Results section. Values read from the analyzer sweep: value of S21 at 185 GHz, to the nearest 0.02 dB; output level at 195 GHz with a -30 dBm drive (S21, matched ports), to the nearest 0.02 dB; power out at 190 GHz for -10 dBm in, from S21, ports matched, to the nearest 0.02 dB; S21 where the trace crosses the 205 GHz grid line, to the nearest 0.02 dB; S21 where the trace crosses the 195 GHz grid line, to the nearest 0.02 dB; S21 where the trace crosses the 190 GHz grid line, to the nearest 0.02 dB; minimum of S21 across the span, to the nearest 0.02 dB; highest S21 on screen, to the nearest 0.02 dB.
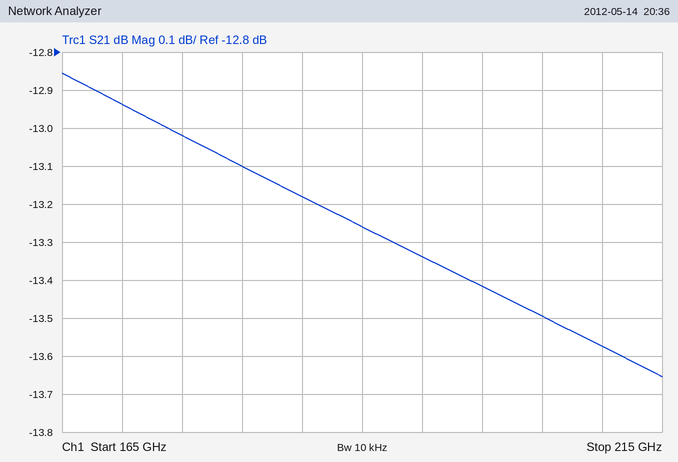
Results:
-13.18 dB
-43.34 dBm
-23.26 dBm
-13.50 dB
-13.34 dB
-13.26 dB
-13.66 dB
-12.86 dB
